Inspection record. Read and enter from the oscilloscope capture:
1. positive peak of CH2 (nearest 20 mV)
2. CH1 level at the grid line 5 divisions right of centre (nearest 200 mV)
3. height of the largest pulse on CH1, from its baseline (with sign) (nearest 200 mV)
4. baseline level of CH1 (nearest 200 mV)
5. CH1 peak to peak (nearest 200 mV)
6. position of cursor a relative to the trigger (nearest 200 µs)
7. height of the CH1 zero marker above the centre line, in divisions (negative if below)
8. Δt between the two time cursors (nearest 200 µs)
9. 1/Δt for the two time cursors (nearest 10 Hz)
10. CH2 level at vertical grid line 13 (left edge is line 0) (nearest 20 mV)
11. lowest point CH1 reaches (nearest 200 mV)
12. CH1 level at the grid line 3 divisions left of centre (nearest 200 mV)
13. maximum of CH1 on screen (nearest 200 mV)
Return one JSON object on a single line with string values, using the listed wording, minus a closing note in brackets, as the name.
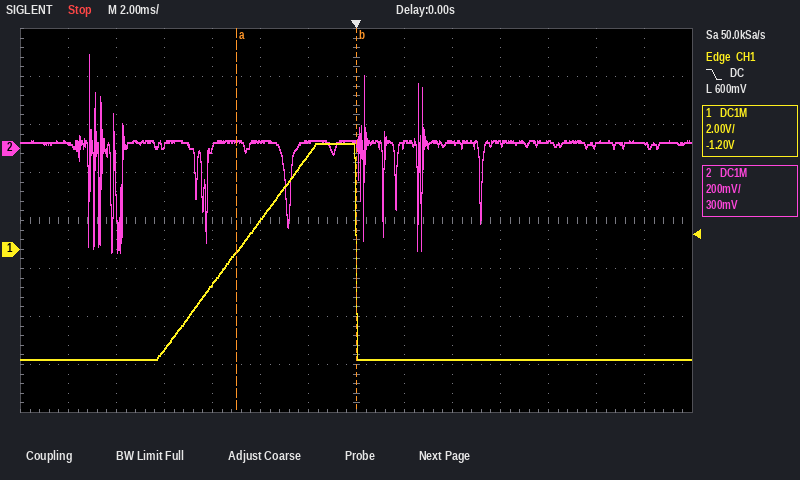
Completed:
{"positive peak of CH2": "400 mV", "CH1 level at the grid line 5 divisions right of centre": "-4.6 V", "height of the largest pulse on CH1, from its baseline (with sign)": "+9.0 V", "baseline level of CH1": "-4.6 V", "CH1 peak to peak": "9.0 V", "position of cursor a relative to the trigger": "-5.0 ms", "height of the CH1 zero marker above the centre line, in divisions": "-0.6 div", "Δt between the two time cursors": "5.0 ms", "1/Δt for the two time cursors": "200 Hz", "CH2 level at vertical grid line 13 (left edge is line 0)": "20 mV", "lowest point CH1 reaches": "-4.6 V", "CH1 level at the grid line 3 divisions left of centre": "-1.4 V", "maximum of CH1 on screen": "4.4 V"}
